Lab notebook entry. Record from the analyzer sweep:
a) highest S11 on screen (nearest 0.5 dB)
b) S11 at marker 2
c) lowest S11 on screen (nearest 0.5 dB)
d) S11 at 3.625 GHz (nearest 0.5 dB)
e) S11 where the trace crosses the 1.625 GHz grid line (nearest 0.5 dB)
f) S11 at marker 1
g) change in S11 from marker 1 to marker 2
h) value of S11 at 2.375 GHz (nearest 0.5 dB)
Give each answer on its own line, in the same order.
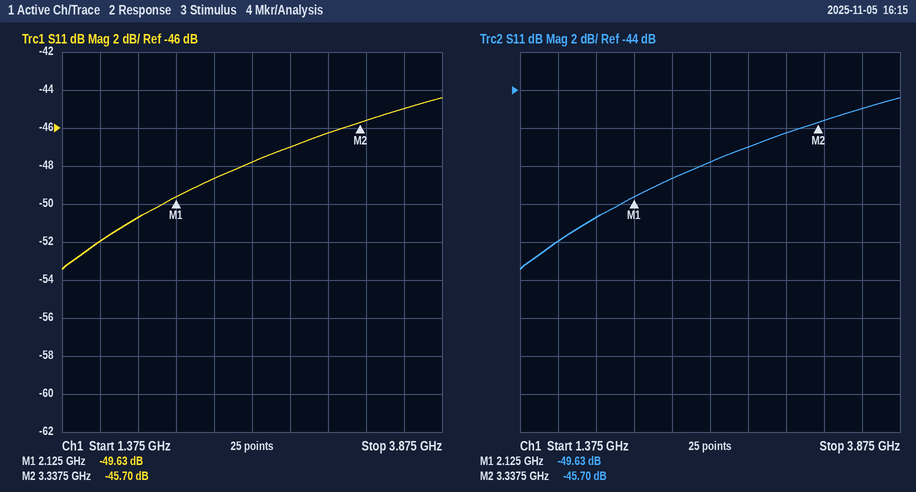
-44.5 dB
-45.70 dB
-53.5 dB
-45.0 dB
-52.0 dB
-49.63 dB
3.93 dB
-48.5 dB
